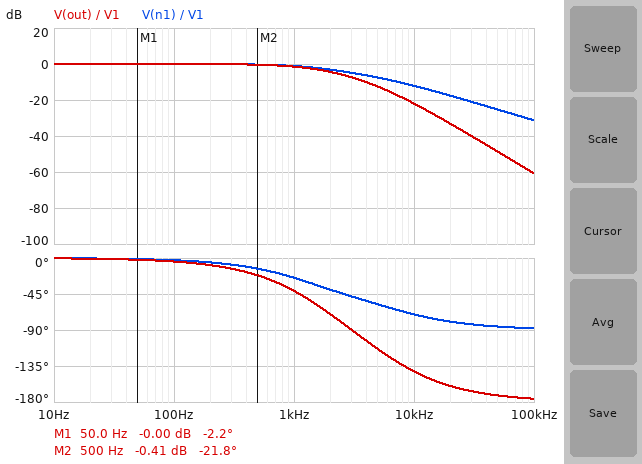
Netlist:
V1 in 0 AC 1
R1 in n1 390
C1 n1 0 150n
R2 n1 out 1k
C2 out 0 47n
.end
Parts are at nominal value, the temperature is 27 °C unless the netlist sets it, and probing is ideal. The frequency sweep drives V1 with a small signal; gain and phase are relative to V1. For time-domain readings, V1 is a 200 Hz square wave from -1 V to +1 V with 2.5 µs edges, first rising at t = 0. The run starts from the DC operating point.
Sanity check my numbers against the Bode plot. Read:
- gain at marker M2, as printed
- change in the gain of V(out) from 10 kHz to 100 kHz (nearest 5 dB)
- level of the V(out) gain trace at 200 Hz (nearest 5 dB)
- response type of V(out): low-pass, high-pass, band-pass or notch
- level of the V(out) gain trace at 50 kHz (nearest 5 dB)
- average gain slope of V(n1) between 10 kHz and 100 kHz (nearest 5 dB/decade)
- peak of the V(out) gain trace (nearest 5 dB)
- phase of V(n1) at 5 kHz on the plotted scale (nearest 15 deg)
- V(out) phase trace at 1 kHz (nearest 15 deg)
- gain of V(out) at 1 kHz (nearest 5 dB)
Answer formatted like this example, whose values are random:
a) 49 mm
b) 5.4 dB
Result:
a) -0.41 dB
b) -40 dB
c) 0 dB
d) low-pass
e) -50 dB
f) -20 dB/decade
g) 0 dB
h) -60 deg
i) -45 deg
j) 0 dB
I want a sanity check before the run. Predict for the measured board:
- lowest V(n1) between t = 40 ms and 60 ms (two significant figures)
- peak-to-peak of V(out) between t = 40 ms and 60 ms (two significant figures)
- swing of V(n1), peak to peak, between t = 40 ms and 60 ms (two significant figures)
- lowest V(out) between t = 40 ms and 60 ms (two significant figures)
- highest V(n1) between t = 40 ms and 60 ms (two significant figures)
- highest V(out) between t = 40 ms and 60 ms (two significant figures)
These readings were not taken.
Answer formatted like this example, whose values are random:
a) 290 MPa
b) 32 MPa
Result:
a) -1.0 V
b) 2.0 V
c) 2.0 V
d) -1.0 V
e) 1.0 V
f) 1.0 V
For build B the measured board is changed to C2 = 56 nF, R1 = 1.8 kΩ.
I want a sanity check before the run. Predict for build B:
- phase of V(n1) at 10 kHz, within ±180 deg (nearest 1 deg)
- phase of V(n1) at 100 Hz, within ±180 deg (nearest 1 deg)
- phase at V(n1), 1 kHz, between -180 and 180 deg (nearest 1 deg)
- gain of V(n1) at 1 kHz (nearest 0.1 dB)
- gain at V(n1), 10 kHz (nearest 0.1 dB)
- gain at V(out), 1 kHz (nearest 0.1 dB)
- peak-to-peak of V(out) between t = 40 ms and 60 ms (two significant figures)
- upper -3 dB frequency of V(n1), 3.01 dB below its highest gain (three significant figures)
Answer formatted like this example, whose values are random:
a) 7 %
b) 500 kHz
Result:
a) -81 deg
b) -13 deg
c) -62 deg
d) -8.2 dB
e) -24.9 dB
f) -8.7 dB
g) 2.0 V
h) 415 Hz
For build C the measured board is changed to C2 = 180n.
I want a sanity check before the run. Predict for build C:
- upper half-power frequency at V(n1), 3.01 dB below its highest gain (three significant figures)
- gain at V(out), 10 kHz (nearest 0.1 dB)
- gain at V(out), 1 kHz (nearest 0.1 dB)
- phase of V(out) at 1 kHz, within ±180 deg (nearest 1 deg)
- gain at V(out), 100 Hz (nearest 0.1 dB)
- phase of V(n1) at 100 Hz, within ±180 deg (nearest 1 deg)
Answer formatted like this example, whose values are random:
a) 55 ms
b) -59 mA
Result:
a) 1.25 kHz
b) -33.1 dB
c) -6.1 dB
d) -73 deg
e) -0.1 dB
f) -5 deg
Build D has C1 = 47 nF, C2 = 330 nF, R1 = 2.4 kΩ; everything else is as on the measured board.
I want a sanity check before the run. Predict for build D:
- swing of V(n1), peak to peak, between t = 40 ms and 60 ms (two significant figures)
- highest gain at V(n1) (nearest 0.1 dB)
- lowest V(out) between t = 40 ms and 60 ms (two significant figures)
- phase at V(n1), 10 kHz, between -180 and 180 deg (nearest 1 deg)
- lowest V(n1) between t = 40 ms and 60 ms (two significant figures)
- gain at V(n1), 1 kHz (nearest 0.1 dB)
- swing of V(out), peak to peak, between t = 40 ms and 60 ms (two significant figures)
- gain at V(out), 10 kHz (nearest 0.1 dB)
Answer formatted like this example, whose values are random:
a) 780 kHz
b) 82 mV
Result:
a) 1.7 V
b) 0 dB
c) -770 mV
d) -65 deg
e) -830 mV
f) -10.6 dB
g) 1.5 V
h) -44.4 dB
